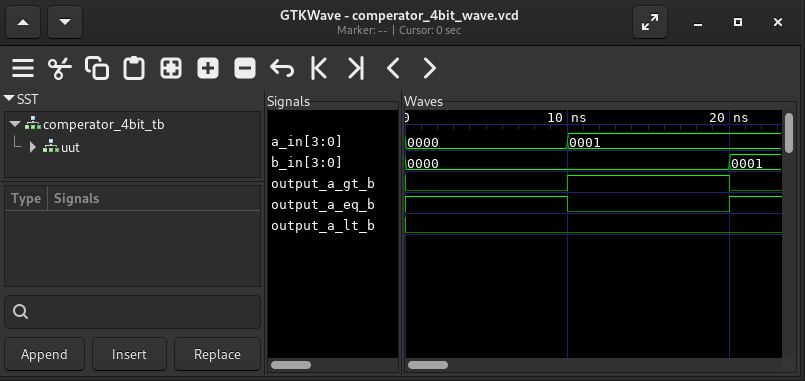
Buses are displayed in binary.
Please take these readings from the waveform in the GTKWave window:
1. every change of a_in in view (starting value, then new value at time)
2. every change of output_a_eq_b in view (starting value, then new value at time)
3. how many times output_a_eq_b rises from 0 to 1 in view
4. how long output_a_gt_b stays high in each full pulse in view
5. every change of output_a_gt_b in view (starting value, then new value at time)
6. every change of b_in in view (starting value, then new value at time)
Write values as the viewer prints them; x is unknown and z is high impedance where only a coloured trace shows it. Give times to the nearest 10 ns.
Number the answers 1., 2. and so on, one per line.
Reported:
1. 0000, 0001 at 10 ns
2. 1, 0 at 10 ns, 1 at 20 ns
3. 1
4. 10 ns
5. 0, 1 at 10 ns, 0 at 20 ns
6. 0000, 0001 at 20 ns
